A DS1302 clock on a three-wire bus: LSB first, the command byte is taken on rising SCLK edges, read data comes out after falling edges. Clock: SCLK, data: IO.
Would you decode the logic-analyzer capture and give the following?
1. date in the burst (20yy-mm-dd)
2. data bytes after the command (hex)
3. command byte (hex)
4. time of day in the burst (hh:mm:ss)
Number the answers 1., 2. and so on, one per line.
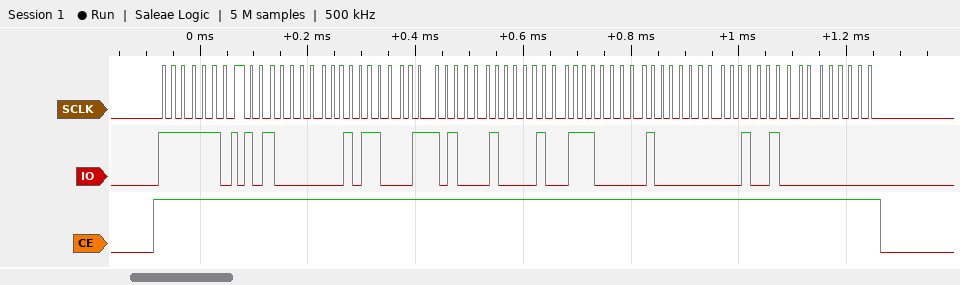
1. 2024-07-21
2. 05 34 16 21 07 01 24 00
3. 0xBF
4. 16:34:05
